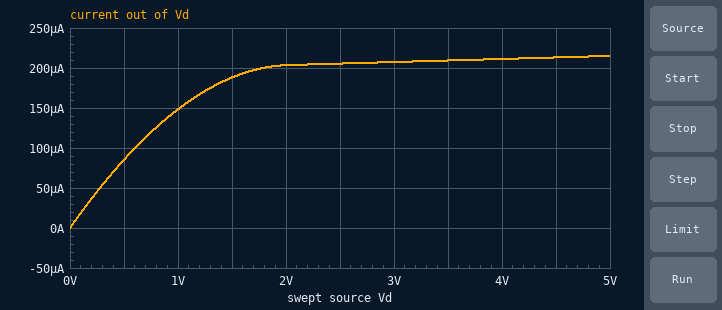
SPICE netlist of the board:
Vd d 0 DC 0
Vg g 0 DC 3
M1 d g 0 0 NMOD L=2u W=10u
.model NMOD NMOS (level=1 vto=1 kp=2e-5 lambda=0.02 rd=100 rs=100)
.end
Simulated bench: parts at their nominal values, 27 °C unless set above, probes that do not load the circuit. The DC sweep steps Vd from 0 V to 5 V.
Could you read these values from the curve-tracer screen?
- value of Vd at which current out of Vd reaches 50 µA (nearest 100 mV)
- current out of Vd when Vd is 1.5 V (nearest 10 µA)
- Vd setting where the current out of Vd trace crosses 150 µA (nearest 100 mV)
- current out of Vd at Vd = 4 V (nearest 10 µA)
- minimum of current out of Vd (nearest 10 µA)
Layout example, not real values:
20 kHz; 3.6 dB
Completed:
300 mV; 190 µA; 1.0 V; 210 µA; 0 A
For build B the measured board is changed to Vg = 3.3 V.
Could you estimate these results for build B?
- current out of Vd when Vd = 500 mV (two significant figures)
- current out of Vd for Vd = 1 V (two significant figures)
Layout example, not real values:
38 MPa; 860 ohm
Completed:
99 µA; 180 µA
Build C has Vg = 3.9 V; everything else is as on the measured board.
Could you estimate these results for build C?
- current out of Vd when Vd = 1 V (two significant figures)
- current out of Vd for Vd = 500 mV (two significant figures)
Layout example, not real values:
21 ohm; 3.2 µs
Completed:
230 µA; 130 µA
